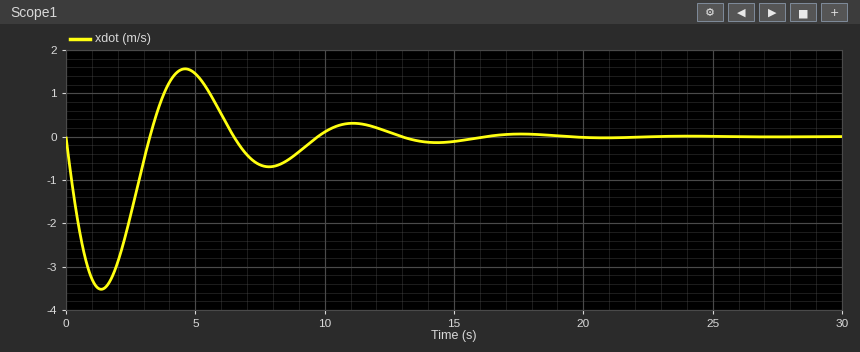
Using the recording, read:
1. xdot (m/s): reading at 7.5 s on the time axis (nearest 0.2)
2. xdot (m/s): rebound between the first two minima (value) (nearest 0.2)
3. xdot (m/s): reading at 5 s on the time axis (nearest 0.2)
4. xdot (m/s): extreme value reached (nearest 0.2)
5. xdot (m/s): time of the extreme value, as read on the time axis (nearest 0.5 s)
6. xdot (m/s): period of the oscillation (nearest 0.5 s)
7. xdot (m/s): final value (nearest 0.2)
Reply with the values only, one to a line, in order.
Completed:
-0.6
1.6
1.4
-3.6
1.5 s
6.5 s
0.0
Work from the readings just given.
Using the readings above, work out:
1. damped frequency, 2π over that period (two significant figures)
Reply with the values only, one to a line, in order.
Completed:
0.97 rad/s
